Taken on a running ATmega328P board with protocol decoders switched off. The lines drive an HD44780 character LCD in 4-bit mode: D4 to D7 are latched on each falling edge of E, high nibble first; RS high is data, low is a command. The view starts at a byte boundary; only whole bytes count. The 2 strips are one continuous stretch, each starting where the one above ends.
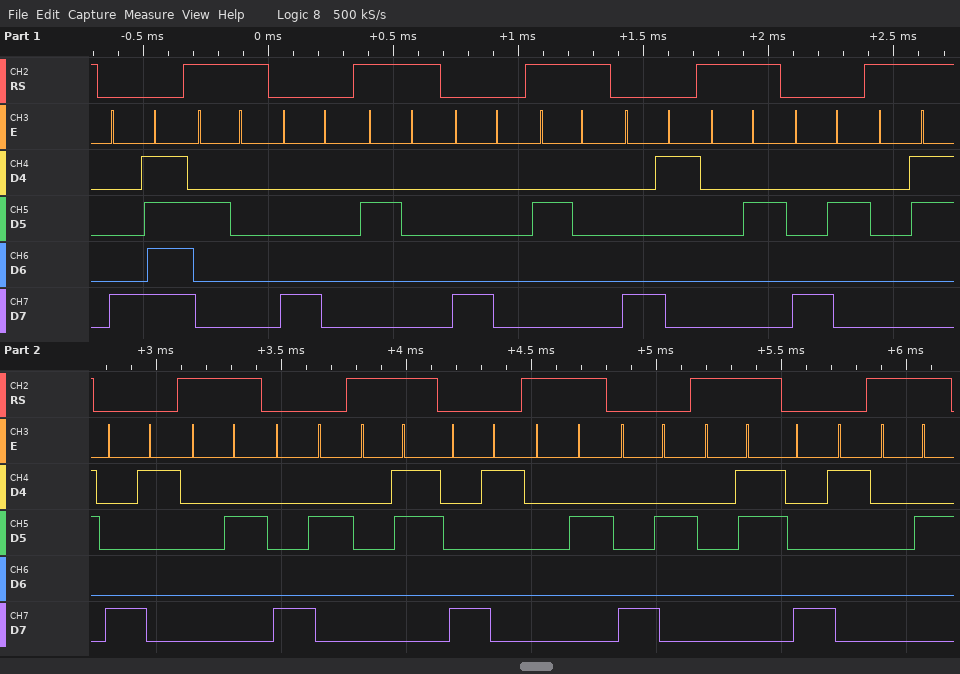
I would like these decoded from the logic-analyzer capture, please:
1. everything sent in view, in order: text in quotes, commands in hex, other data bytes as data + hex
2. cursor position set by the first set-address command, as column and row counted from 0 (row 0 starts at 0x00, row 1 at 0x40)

0x8F " " 0x80 " " 0x80 " " 0x81 data 02 0x82 data 03 0x81 data 02 0x82 data 03 0x81 data 02 0x82 data 03 0x81 data 02
column 15, row 0
